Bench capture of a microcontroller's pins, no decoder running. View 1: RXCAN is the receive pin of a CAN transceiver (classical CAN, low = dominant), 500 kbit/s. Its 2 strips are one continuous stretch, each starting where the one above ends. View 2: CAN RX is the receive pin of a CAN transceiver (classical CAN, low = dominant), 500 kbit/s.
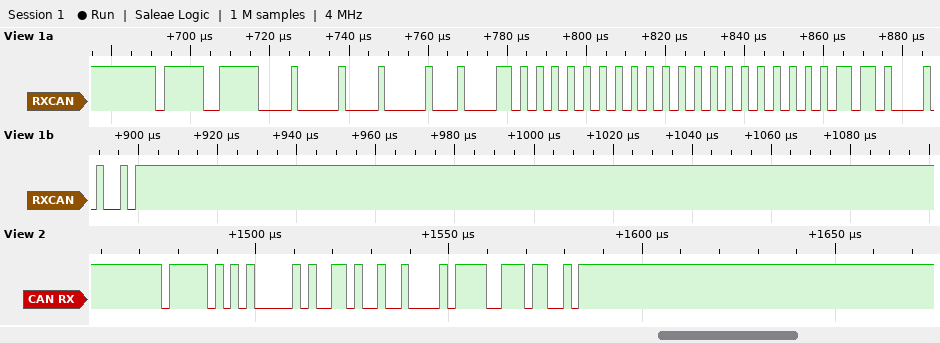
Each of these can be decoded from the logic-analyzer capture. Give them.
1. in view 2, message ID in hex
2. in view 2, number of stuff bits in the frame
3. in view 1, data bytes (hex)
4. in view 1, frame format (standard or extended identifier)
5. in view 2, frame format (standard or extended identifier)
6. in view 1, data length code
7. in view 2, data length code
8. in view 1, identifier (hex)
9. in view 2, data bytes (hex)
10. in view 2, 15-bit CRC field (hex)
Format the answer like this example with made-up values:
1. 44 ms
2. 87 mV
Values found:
1. 0x7EA
2. 2
3. 02 01 0D 55 55 55 55 55
4. standard
5. standard
6. 8
7. 2
8. 0x7DF
9. 69 21
10. 0x3CEC
